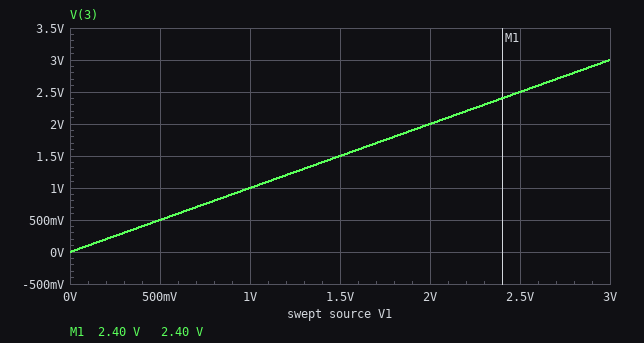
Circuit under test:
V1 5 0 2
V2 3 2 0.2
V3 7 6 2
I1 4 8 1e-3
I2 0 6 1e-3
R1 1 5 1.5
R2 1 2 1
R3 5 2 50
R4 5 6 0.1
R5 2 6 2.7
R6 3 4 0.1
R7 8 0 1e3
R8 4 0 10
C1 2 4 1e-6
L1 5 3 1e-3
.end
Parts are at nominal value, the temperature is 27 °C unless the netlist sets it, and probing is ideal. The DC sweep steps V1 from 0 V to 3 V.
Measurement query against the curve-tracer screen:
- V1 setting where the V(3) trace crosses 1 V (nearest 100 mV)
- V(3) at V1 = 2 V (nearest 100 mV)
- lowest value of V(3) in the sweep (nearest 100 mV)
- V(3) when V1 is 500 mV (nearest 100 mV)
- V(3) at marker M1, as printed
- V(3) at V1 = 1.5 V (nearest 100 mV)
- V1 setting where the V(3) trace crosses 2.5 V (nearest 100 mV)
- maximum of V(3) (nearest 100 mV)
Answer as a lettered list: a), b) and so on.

a) 1.0 V
b) 2.0 V
c) 0 V
d) 500 mV
e) 2.40 V
f) 1.5 V
g) 2.5 V
h) 3.0 V
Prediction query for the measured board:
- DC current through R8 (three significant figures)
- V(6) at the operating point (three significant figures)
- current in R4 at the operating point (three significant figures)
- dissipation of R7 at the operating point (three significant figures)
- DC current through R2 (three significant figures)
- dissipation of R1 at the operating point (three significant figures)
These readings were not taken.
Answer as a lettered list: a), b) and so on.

a) 198 mA
b) 1.99 V
c) 70.5 mA
d) 1.00 mW
e) 80.0 mA
f) 9.60 mW
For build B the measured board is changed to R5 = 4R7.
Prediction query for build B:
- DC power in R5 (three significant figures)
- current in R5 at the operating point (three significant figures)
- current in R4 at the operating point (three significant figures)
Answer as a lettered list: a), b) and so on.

a) 8.17 mW
b) 41.7 mA
c) 40.7 mA
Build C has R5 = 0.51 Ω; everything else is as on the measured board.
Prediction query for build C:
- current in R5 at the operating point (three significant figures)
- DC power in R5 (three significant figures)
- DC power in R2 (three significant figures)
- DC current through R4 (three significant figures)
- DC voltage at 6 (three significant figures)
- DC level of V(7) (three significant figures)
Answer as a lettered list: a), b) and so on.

a) 328 mA
b) 54.9 mW
c) 6.40 mW
d) 327 mA
e) 1.97 V
f) 3.97 V
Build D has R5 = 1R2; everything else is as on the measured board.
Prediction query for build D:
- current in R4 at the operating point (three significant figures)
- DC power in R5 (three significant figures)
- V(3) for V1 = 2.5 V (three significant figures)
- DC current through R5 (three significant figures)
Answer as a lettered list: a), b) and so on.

a) 153 mA
b) 28.4 mW
c) 2.50 V
d) 154 mA
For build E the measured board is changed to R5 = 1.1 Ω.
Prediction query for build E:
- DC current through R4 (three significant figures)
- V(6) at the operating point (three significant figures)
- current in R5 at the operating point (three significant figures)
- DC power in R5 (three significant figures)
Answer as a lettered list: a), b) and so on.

a) 166 mA
b) 1.98 V
c) 167 mA
d) 30.6 mW
